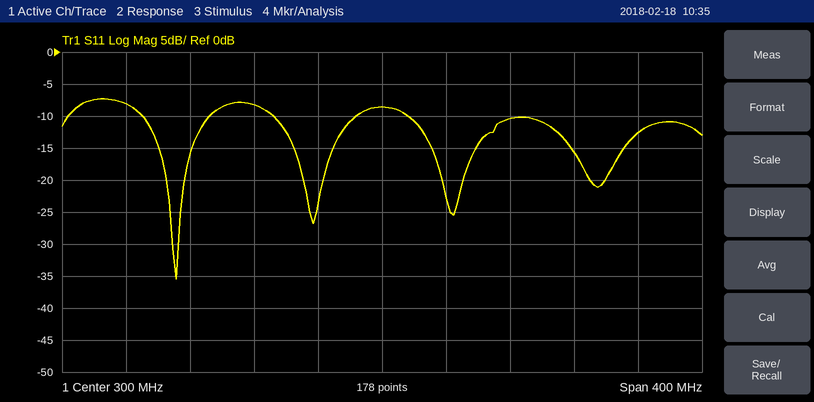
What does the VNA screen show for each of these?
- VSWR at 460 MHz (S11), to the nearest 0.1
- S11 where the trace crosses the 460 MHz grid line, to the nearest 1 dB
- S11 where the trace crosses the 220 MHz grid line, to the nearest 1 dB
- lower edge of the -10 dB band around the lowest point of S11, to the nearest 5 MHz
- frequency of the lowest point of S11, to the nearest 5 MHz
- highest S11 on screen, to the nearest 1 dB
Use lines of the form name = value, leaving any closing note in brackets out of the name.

VSWR at 460 MHz (S11), to the nearest 0.1 = 1.6
S11 where the trace crosses the 460 MHz grid line, to the nearest 1 dB = -13 dB
S11 where the trace crosses the 220 MHz grid line, to the nearest 1 dB = -8 dB
lower edge of the -10 dB band around the lowest point of S11, to the nearest 5 MHz = 150 MHz
frequency of the lowest point of S11, to the nearest 5 MHz = 170 MHz
highest S11 on screen, to the nearest 1 dB = -7 dB
